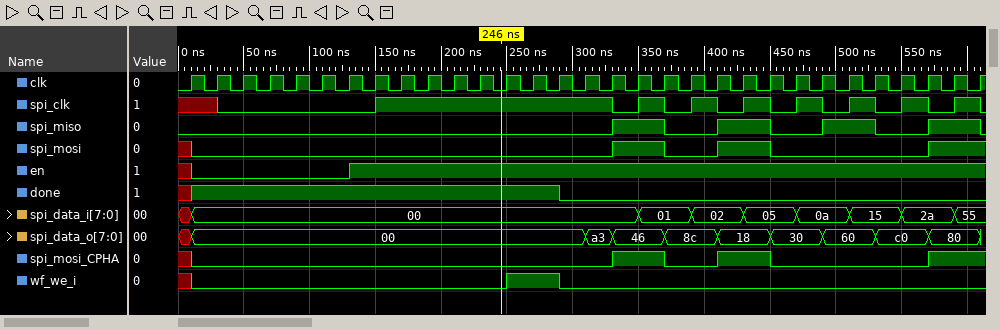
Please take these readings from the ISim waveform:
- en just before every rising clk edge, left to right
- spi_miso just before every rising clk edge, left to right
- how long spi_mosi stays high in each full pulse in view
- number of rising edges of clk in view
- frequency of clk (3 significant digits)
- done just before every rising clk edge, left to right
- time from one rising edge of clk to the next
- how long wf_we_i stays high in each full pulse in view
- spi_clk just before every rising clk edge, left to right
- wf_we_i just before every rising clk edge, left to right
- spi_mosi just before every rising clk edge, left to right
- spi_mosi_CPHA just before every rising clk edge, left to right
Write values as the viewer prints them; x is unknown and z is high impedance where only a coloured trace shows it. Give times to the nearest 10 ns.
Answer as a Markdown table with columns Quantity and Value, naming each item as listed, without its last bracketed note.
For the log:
| Quantity | Value |
|---|---|
| en just before every rising clk edge, left to right | x 0 0 0 0 0 0 1 1 1 1 1 1 1 1 1 1 1 1 1 1 1 1 1 1 1 1 1 1 1 1 |
| spi_miso just before every rising clk edge, left to right | 0 0 0 0 0 0 0 0 0 0 0 0 0 0 0 0 0 1 1 0 0 1 1 0 0 1 1 0 0 1 1 |
| how long spi_mosi stays high in each full pulse in view | 40 ns, 40 ns |
| number of rising edges of clk in view | 31 |
| frequency of clk | 50.0 MHz |
| done just before every rising clk edge, left to right | x 1 1 1 1 1 1 1 1 1 1 1 1 1 1 0 0 0 0 0 0 0 0 0 0 0 0 0 0 0 0 |
| time from one rising edge of clk to the next | 20 ns |
| how long wf_we_i stays high in each full pulse in view | 40 ns |
| spi_clk just before every rising clk edge, left to right | x x 0 0 0 0 0 0 1 1 1 1 1 1 1 1 1 0 1 0 1 0 1 0 1 0 1 0 1 0 1 |
| wf_we_i just before every rising clk edge, left to right | x 0 0 0 0 0 0 0 0 0 0 0 0 1 1 0 0 0 0 0 0 0 0 0 0 0 0 0 0 0 0 |
| spi_mosi just before every rising clk edge, left to right | x 0 0 0 0 0 0 0 0 0 0 0 0 0 0 0 0 1 1 0 0 1 1 0 0 0 0 0 0 1 1 |
| spi_mosi_CPHA just before every rising clk edge, left to right | x 0 0 0 0 0 0 0 0 0 0 0 0 0 0 0 0 1 1 0 0 1 1 0 0 0 0 0 0 1 1 |
